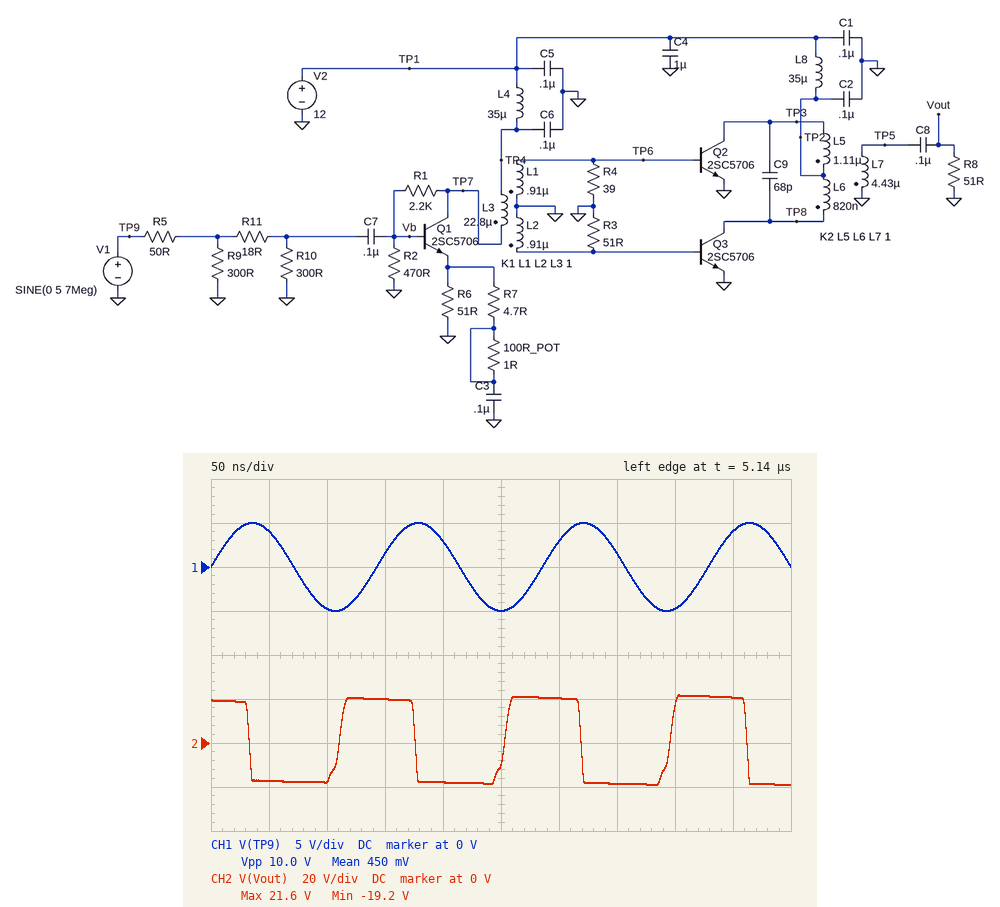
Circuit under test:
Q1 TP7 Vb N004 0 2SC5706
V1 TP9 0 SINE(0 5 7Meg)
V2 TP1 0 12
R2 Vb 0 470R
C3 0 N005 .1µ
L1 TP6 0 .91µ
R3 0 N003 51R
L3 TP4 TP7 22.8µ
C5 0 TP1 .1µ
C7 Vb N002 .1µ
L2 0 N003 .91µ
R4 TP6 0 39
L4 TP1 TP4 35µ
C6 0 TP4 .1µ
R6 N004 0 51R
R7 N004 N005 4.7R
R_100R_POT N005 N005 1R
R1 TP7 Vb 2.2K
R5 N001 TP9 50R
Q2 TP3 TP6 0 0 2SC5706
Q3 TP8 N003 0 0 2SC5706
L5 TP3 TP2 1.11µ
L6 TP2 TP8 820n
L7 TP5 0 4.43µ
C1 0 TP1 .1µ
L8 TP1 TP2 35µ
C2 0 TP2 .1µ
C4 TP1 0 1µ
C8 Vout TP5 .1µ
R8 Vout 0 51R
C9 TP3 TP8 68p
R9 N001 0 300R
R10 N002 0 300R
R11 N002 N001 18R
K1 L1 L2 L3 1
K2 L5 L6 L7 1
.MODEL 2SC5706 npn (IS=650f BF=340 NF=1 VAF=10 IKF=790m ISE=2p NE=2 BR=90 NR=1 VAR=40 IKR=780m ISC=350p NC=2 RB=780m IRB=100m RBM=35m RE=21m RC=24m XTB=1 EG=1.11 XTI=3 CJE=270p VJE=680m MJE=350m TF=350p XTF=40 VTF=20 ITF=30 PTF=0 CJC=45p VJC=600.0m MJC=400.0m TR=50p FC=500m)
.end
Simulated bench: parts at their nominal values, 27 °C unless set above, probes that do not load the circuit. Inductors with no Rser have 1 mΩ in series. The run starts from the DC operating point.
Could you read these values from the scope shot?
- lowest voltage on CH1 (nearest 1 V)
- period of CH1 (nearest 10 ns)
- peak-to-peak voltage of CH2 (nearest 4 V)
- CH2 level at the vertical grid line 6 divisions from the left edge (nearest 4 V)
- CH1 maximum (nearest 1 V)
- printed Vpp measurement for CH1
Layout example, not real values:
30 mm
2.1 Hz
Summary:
-5 V
140 ns
40 V
20 V
5 V
10.0 V
